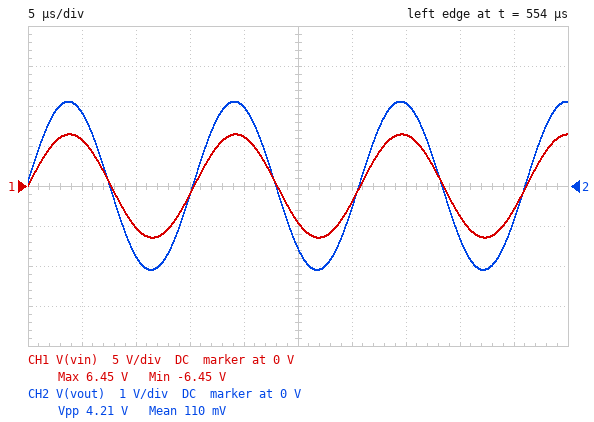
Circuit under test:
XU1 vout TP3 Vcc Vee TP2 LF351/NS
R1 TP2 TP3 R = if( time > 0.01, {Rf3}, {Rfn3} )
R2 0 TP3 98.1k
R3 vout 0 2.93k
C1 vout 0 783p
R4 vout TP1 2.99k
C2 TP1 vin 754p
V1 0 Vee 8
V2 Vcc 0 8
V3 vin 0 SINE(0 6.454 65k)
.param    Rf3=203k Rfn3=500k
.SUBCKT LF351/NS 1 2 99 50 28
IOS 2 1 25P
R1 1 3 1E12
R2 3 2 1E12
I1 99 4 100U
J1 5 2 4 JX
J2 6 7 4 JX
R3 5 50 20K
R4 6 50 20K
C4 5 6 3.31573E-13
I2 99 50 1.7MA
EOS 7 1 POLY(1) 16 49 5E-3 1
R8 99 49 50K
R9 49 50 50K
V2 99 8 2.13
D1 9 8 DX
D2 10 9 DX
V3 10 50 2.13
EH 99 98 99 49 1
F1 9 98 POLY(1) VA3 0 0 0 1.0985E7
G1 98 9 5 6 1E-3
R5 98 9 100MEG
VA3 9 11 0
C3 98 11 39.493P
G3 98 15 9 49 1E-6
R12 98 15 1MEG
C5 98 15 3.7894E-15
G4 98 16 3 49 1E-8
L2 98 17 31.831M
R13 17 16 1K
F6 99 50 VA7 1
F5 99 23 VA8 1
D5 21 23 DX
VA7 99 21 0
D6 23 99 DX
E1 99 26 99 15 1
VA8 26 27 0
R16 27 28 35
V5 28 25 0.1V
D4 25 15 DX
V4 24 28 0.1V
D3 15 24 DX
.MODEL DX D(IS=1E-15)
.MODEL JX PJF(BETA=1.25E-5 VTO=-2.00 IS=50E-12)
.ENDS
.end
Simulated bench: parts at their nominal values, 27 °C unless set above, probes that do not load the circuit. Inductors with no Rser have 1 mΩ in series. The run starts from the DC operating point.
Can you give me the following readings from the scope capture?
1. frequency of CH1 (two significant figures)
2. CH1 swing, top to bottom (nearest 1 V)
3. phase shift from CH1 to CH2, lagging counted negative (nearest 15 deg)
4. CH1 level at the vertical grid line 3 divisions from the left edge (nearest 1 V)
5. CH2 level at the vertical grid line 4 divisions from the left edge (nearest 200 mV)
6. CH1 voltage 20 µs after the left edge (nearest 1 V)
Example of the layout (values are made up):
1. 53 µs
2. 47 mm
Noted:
1. 65 kHz
2. 13 V
3. 0 deg
4. -1 V
5. 2.0 V
6. 6 V
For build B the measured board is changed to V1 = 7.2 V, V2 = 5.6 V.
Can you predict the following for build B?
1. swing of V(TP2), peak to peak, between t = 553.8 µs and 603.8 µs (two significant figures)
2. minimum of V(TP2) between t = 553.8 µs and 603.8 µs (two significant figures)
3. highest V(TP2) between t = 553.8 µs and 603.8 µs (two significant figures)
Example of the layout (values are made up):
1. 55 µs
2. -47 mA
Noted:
1. 10 V
2. -5.8 V
3. 4.2 V
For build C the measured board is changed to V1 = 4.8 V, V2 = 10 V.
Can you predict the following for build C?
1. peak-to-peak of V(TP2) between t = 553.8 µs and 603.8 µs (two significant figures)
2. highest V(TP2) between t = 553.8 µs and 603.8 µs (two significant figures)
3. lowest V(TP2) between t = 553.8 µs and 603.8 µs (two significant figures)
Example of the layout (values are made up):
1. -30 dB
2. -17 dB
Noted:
1. 12 V
2. 8.6 V
3. -3.4 V
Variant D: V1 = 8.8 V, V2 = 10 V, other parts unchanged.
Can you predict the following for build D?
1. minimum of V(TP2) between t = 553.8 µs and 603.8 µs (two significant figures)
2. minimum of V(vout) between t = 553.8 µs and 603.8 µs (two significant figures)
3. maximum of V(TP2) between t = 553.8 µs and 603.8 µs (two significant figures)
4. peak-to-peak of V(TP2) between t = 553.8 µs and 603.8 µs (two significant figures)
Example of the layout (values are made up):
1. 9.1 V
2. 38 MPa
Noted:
1. -7.4 V
2. -2.1 V
3. 8.6 V
4. 16 V
